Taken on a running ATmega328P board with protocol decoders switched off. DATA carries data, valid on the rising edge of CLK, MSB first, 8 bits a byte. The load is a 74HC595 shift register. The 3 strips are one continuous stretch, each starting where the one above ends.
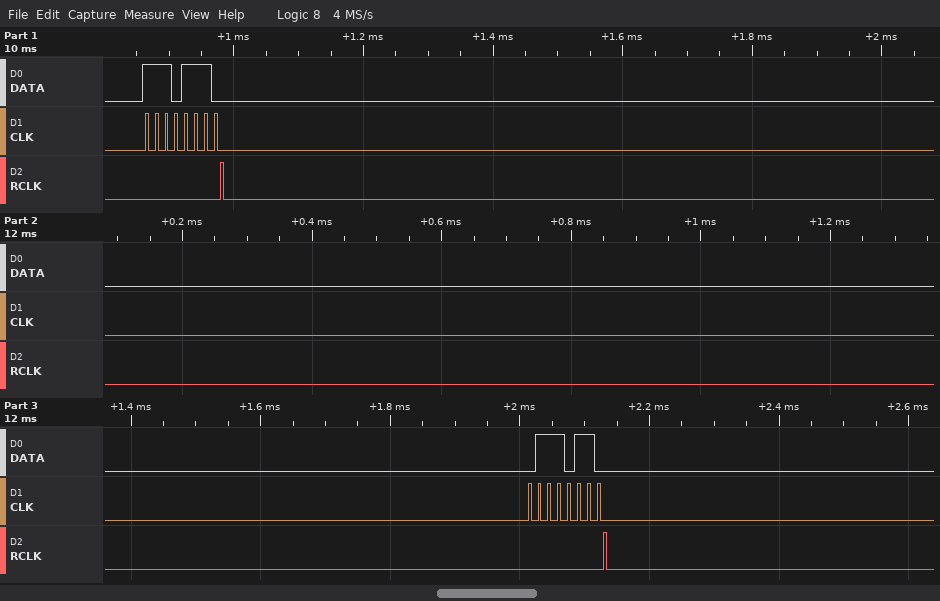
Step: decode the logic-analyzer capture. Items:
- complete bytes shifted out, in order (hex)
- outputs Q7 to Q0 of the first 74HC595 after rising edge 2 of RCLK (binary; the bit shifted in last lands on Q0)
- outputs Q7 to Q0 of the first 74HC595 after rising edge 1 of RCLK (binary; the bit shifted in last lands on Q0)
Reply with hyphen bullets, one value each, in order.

- EE 76
- 01110110
- 11101110
